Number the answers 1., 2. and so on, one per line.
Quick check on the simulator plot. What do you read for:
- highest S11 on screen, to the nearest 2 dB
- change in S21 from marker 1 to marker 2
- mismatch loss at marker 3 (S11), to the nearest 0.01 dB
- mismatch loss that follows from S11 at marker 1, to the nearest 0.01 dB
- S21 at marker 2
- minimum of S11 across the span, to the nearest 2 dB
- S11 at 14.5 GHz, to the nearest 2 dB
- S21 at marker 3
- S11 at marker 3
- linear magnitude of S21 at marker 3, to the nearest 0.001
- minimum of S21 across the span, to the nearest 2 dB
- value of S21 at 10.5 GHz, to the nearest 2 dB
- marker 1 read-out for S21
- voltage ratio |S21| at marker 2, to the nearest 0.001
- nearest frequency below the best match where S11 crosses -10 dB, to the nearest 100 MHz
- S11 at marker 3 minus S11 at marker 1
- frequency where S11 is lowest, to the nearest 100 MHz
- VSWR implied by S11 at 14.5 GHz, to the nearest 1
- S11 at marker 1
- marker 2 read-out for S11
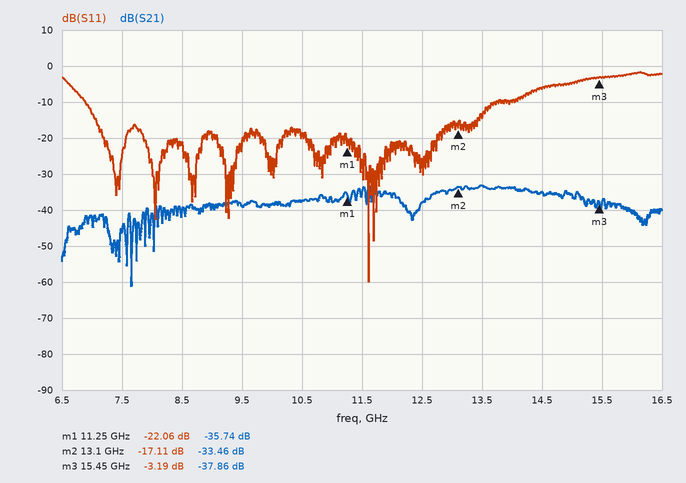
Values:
1. -2 dB
2. 2.28 dB
3. 2.84 dB
4. 0.03 dB
5. -33.46 dB
6. -60 dB
7. -6 dB
8. -37.86 dB
9. -3.19 dB
10. 0.013
11. -62 dB
12. -38 dB
13. -35.74 dB
14. 0.021
15. 6.9 GHz
16. 18.87 dB
17. 11.6 GHz
18. 3
19. -22.06 dB
20. -17.11 dB
